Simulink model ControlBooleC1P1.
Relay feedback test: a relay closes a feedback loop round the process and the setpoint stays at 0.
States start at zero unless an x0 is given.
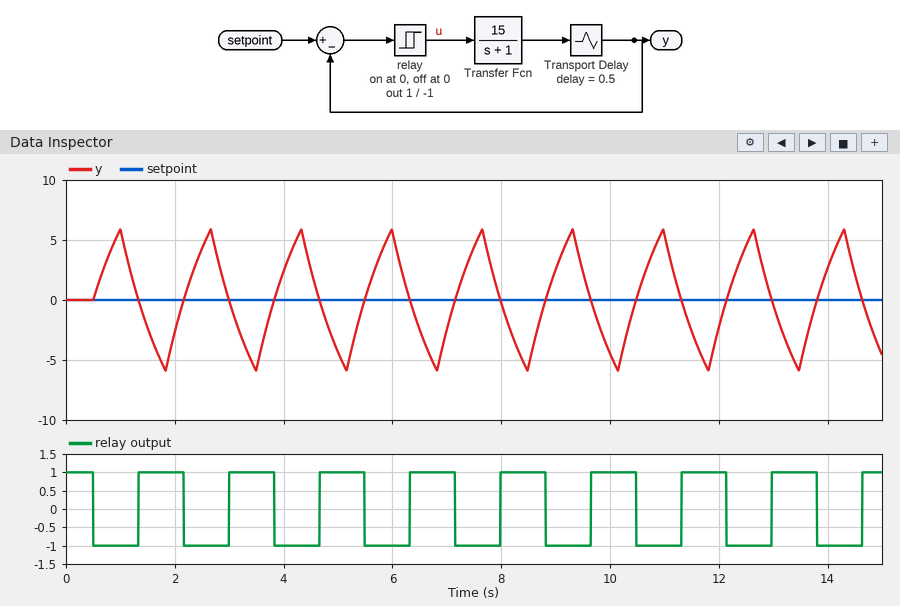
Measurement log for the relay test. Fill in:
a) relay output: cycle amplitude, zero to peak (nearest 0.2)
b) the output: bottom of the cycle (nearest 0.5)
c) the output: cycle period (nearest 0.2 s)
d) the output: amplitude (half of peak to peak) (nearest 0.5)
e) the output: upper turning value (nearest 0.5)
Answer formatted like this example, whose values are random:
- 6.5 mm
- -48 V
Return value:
- 1.0
- -6.0
- 1.6 s
- 6.0
- 6.0
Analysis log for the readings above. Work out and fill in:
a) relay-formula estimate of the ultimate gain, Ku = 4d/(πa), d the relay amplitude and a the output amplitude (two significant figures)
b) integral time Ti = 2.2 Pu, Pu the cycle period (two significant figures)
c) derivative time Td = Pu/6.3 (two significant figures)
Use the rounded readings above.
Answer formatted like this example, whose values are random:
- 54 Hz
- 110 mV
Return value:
- 0.21
- 3.5 s
- 0.25 s
